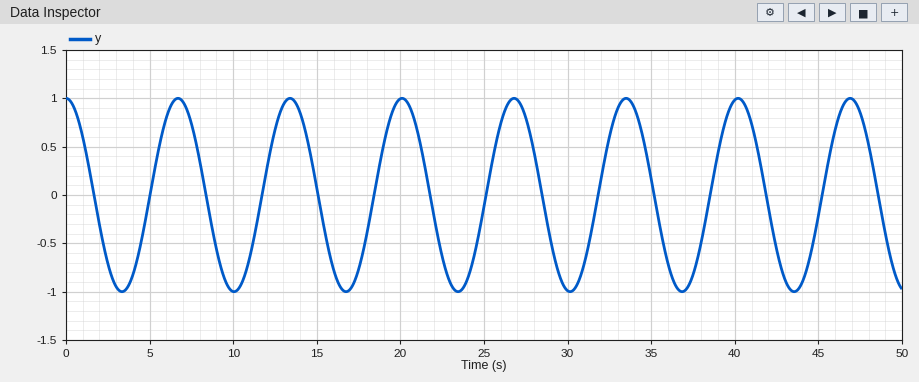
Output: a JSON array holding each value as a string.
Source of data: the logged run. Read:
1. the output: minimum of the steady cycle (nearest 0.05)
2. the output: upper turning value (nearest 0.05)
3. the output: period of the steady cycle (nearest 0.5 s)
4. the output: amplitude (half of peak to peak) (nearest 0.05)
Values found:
["-1.00", "1.00", "6.5 s", "1.00"]
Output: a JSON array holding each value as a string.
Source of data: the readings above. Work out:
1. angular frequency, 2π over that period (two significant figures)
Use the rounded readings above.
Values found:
["0.97 rad/s"]
